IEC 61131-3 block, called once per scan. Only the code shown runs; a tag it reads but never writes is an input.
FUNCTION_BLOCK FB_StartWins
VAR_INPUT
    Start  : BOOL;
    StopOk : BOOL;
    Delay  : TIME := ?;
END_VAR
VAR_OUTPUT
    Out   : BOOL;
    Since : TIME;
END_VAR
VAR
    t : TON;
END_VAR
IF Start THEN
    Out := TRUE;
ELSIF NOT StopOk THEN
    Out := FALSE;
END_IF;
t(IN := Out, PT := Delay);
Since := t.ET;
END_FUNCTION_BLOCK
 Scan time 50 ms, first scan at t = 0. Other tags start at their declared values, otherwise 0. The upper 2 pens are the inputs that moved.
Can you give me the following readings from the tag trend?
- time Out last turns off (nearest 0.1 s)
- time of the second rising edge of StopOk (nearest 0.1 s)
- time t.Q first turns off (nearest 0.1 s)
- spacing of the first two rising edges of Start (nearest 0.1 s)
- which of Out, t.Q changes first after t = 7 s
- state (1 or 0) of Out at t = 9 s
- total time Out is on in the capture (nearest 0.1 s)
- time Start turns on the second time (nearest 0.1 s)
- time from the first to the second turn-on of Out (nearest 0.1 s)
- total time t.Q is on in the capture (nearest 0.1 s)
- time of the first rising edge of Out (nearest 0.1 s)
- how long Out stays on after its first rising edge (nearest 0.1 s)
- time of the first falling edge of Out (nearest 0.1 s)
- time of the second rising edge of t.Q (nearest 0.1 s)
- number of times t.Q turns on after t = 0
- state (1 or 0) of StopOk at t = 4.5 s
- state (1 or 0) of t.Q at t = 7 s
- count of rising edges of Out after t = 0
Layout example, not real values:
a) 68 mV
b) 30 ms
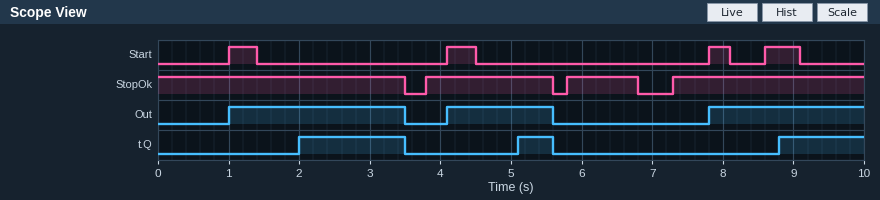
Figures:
a) 5.6 s
b) 5.8 s
c) 3.5 s
d) 3.1 s
e) Out
f) 1
g) 6.2 s
h) 4.1 s
i) 3.1 s
j) 3.2 s
k) 1.0 s
l) 2.5 s
m) 3.5 s
n) 5.1 s
o) 3
p) 1
q) 0
r) 3
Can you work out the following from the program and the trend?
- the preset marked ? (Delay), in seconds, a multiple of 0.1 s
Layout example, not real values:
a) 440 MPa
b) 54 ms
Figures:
a) 1.0 s
